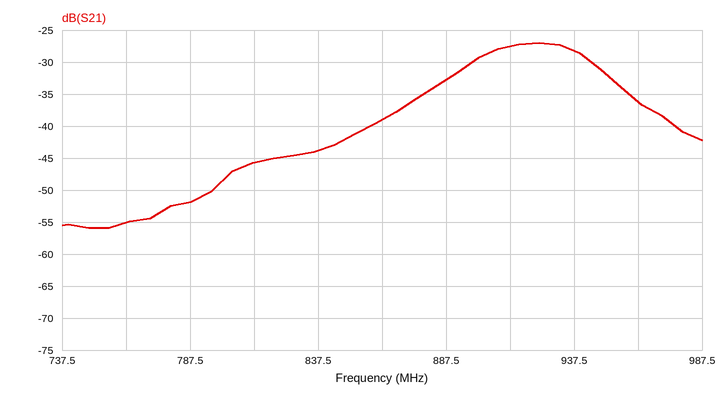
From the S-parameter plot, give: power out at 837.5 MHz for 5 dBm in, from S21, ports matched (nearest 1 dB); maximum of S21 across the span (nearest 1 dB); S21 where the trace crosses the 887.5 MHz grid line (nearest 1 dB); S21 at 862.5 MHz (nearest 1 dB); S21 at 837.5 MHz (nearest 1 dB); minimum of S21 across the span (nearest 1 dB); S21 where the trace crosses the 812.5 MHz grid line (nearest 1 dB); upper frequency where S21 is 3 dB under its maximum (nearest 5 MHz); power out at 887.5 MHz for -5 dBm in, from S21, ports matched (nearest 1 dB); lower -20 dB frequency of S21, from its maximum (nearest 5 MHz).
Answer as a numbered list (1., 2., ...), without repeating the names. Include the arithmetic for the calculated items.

1. 5 dBm + (-44 dB) = -39 dBm
2. -27 dB
3. -33 dB
4. -39 dB
5. -44 dB
6. -56 dB
7. -46 dB
8. 945 MHz
9. -5 dBm + (-33 dB) = -38 dBm
10. 805 MHz
